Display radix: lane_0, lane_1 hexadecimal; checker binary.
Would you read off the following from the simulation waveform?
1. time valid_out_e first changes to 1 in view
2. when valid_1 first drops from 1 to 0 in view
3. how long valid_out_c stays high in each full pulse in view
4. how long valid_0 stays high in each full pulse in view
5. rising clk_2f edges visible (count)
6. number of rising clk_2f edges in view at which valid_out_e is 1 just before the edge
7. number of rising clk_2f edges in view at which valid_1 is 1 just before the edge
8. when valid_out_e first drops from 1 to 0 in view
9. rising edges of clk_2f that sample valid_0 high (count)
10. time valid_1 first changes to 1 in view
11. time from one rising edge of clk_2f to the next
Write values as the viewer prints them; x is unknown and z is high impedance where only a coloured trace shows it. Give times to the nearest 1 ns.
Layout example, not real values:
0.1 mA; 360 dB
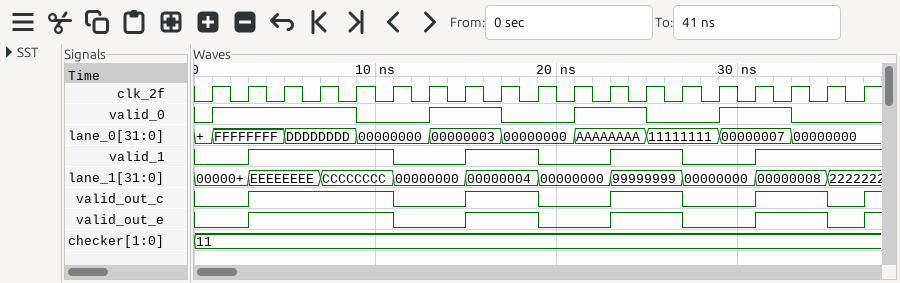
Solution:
3 ns; 11 ns; 8 ns, 4 ns, 4 ns, 4 ns; 8 ns, 4 ns, 4 ns, 4 ns; 19; 10; 11; 11 ns; 10; 3 ns; 2 ns
